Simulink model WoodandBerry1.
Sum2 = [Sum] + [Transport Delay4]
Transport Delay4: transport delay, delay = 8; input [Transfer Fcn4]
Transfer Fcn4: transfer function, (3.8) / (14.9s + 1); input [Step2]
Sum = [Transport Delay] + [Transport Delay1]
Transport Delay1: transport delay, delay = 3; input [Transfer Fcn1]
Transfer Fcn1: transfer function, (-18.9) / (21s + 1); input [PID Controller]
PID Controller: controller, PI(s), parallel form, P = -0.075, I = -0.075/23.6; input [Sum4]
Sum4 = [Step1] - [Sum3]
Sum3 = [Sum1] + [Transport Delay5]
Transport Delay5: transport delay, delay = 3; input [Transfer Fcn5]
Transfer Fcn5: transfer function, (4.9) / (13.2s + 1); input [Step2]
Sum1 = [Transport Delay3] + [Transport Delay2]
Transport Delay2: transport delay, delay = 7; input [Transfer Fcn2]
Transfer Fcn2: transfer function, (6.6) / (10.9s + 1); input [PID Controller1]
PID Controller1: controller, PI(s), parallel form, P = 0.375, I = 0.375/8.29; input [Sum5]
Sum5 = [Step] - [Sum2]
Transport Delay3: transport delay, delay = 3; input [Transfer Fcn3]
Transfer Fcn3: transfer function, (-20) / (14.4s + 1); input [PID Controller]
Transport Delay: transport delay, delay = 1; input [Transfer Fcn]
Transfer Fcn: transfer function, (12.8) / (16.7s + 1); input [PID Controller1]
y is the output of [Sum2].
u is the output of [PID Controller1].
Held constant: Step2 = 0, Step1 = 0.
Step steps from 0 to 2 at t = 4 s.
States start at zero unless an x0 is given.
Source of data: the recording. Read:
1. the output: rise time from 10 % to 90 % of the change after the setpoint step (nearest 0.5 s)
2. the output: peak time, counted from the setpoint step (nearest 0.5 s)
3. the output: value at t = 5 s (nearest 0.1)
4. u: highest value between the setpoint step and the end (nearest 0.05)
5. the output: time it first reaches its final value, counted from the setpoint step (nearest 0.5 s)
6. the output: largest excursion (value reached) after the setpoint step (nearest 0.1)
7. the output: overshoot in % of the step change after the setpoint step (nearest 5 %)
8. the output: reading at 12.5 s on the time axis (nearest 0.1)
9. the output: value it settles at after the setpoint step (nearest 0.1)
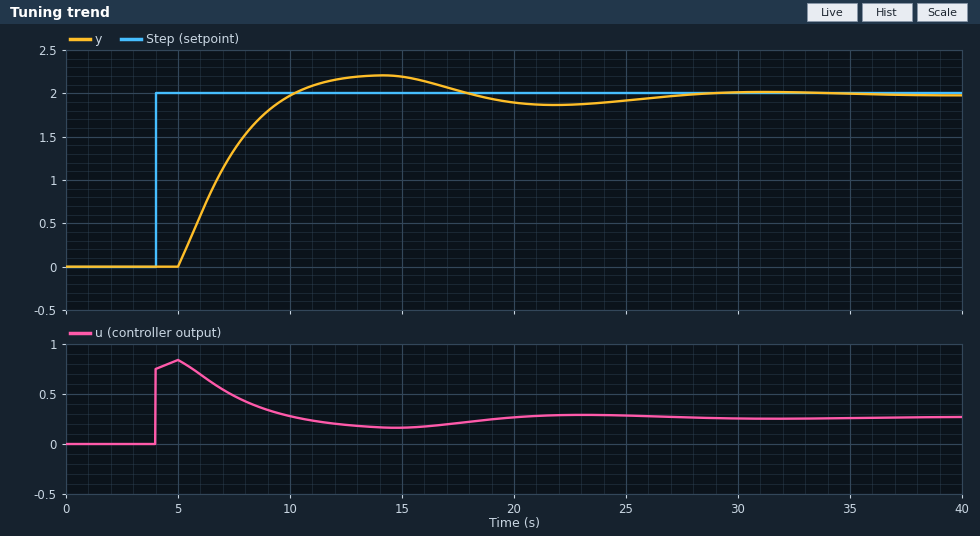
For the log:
3.5 s
10.0 s
0.0
0.85
6.0 s
2.2
10 %
2.2
2.0
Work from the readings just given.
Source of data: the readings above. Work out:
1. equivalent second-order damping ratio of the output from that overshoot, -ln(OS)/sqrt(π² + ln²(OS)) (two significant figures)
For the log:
0.59
